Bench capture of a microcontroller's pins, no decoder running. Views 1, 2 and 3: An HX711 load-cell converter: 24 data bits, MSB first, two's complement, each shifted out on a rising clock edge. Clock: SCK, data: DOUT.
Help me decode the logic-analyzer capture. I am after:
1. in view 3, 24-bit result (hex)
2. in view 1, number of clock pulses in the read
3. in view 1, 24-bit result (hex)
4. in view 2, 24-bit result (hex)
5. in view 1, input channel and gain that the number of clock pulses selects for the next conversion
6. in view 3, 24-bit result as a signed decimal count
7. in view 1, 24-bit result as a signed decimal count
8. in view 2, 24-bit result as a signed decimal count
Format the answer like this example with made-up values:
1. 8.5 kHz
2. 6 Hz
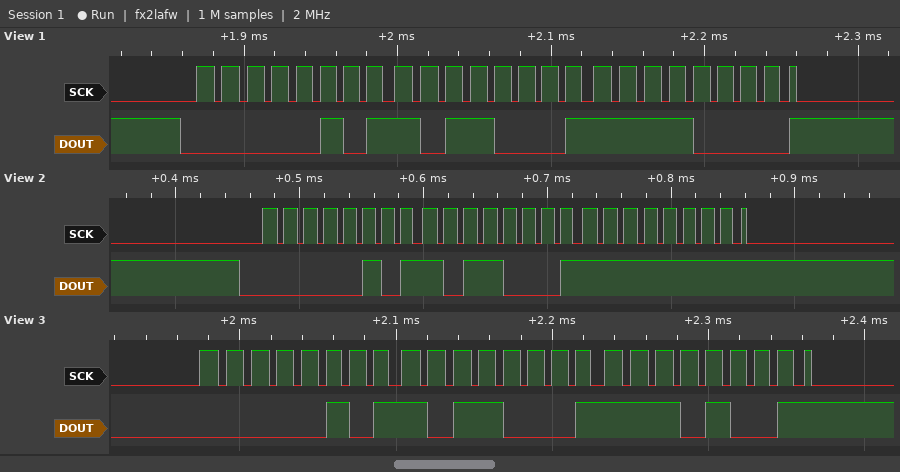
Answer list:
1. 0x05B1E9
2. 25
3. 0x05B1F0
4. 0x05B1FF
5. channel A, gain 128
6. 373225
7. 373232
8. 373247
